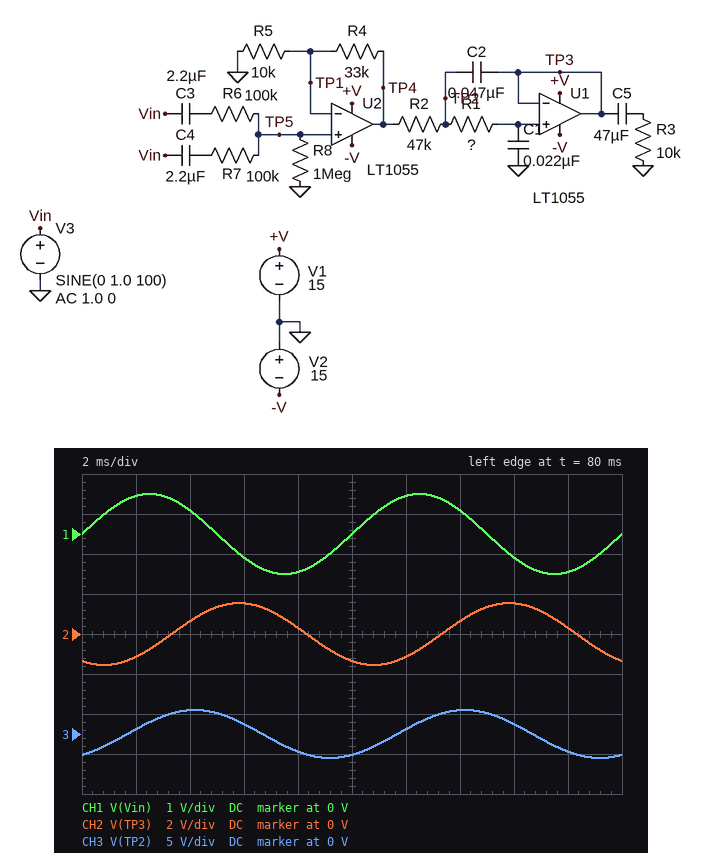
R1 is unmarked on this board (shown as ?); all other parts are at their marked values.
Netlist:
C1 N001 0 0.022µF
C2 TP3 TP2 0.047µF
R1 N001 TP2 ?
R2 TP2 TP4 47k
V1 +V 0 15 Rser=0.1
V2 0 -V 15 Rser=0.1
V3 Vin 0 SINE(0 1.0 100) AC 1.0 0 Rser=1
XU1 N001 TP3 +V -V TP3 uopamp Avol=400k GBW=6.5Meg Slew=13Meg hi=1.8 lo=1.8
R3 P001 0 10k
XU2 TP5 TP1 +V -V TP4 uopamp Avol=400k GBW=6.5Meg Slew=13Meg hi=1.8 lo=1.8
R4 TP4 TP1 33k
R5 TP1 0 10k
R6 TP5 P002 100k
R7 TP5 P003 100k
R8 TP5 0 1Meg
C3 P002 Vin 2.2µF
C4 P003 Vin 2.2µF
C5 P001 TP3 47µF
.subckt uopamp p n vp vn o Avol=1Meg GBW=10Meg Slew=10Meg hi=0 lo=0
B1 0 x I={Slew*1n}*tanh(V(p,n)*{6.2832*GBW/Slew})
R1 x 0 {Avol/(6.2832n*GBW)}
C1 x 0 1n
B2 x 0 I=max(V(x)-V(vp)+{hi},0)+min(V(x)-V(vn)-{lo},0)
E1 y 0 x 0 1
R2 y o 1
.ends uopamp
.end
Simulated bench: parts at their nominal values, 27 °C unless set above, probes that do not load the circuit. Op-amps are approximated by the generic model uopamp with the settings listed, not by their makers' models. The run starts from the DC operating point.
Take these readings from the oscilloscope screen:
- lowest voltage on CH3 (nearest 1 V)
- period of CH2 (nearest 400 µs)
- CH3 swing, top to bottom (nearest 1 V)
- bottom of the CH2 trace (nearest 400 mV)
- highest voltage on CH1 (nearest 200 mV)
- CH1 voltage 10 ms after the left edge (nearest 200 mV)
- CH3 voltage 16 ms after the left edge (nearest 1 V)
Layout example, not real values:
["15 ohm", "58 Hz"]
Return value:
["-3 V", "10.0 ms", "6 V", "-1.6 V", "1.0 V", "0 V", "1 V"]
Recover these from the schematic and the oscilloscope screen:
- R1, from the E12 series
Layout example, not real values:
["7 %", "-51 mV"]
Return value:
["120 kΩ"]
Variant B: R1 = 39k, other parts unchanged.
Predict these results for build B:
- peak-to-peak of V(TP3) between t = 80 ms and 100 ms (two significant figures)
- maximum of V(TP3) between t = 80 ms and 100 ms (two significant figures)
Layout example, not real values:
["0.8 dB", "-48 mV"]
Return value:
["6.7 V", "3.4 V"]
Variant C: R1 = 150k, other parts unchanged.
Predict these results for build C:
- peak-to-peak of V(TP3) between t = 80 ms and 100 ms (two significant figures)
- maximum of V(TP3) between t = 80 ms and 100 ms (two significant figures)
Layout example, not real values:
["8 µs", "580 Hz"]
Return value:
["2.5 V", "1.2 V"]
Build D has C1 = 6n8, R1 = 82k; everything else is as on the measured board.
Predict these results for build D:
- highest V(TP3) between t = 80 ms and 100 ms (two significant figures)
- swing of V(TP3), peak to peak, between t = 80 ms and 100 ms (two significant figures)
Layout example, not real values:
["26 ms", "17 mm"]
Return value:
["5.4 V", "11 V"]
